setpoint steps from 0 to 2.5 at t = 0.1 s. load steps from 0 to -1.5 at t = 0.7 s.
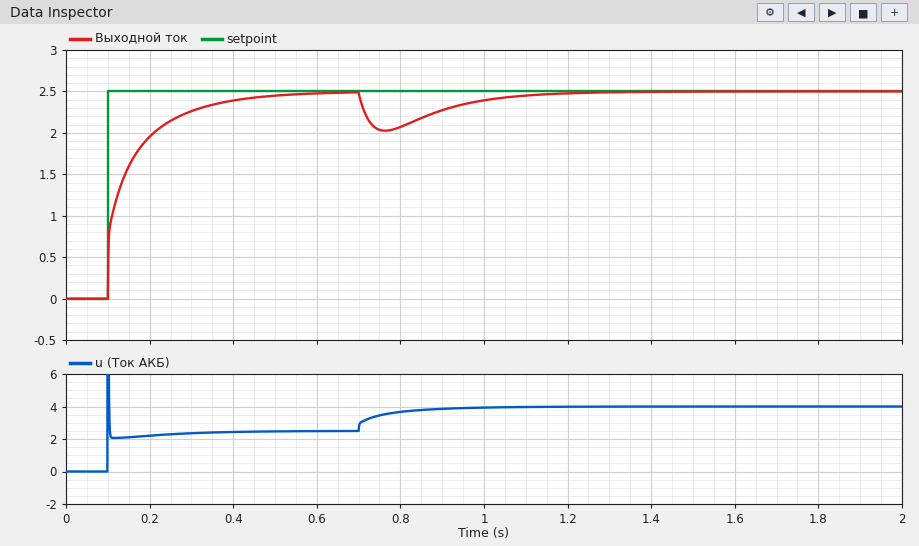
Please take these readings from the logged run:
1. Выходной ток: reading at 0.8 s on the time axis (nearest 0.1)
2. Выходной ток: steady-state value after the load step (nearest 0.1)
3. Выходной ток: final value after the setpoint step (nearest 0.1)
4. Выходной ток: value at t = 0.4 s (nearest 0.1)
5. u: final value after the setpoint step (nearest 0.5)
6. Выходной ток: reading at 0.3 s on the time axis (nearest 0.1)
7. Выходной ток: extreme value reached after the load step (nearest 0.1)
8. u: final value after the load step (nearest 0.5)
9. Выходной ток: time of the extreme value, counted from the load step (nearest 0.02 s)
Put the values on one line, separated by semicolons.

2.1; 2.5; 2.5; 2.4; 2.5; 2.3; 2.0; 4.0; 0.06 s
